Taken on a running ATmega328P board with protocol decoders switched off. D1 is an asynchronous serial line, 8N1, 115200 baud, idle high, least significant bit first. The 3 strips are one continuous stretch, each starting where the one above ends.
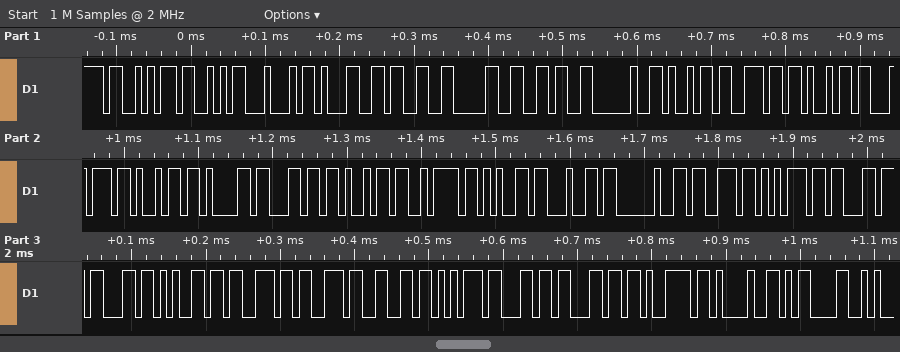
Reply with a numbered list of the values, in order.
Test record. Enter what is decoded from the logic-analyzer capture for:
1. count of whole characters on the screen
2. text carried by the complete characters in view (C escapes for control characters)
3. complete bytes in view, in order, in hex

1. 34
2. "SSD1306 initialized successfully!\r"
3. 53 53 44 31 33 30 36 20 69 6E 69 74 69 61 6C 69 7A 65 64 20 73 75 63 63 65 73 73 66 75 6C 6C 79 21 0D
